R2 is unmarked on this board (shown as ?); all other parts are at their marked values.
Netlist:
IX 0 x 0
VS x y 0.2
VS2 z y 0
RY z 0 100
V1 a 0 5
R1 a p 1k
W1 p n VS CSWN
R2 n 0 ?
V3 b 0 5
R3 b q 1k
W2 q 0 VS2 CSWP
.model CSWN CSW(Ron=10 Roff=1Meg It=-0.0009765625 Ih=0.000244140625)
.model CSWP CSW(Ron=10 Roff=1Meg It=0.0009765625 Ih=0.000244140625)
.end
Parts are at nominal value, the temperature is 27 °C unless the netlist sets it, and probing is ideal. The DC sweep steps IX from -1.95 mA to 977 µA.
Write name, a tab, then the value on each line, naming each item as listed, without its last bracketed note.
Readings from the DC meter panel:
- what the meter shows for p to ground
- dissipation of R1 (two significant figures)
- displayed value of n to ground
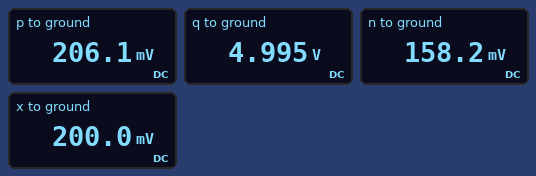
what the meter shows for p to ground	206.1 mV
dissipation of R1	23 mW
displayed value of n to ground	158.2 mV
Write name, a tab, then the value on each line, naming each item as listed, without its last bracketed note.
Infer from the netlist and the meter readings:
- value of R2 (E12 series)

value of R2	33 Ω
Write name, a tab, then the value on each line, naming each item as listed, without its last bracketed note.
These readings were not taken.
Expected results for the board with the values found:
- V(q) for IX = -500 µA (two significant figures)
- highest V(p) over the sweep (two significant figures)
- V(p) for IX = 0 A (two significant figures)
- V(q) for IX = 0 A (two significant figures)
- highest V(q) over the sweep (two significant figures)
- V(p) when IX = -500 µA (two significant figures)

V(q) for IX = -500 µA	5.0 V
highest V(p) over the sweep	5.0 V
V(p) for IX = 0 A	210 mV
V(q) for IX = 0 A	5.0 V
highest V(q) over the sweep	5.0 V
V(p) when IX = -500 µA	210 mV
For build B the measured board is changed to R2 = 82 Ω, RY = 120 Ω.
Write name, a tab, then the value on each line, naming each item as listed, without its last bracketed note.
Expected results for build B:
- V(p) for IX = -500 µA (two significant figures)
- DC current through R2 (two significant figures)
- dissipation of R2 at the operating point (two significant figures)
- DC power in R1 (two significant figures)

V(p) for IX = -500 µA	420 mV
DC current through R2	4.6 mA
dissipation of R2 at the operating point	1.7 mW
DC power in R1	21 mW
